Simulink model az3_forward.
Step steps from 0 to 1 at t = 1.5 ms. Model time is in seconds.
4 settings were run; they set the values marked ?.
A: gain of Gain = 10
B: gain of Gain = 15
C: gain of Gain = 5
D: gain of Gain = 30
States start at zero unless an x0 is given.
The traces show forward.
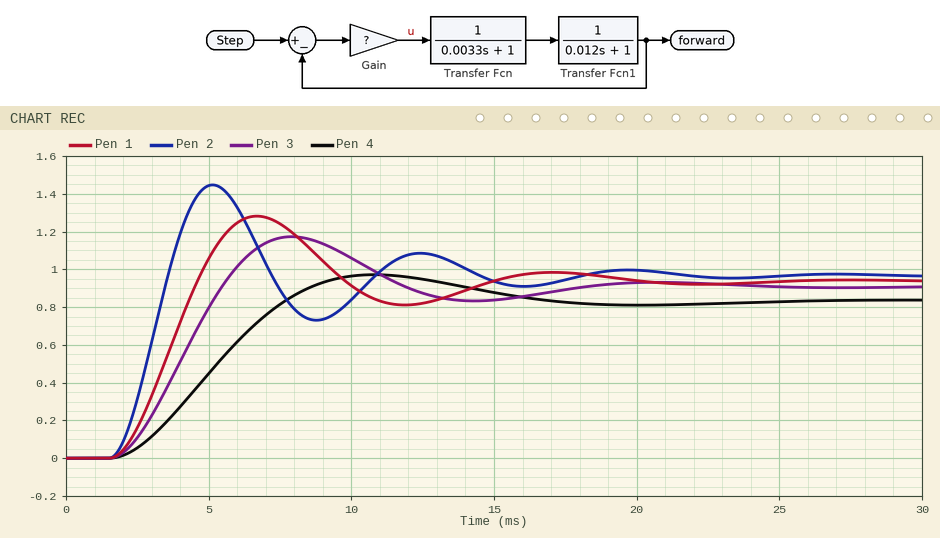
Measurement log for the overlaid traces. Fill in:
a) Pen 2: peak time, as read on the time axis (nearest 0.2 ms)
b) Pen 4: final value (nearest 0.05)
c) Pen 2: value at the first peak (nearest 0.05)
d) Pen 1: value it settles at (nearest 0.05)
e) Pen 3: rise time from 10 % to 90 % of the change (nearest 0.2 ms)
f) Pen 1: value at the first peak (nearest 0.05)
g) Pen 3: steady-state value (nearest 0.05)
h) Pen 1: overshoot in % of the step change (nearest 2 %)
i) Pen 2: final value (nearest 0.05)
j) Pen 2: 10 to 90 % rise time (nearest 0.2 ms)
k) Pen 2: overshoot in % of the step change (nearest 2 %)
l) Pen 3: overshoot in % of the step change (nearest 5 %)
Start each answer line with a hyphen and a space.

- 5.2 ms
- 0.85
- 1.45
- 0.95
- 2.6 ms
- 1.30
- 0.90
- 36 %
- 0.95
- 1.4 ms
- 50 %
- 30 %
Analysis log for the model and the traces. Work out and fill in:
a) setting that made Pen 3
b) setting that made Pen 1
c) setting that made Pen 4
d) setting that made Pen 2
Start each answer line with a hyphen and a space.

- A
- B
- C
- D
